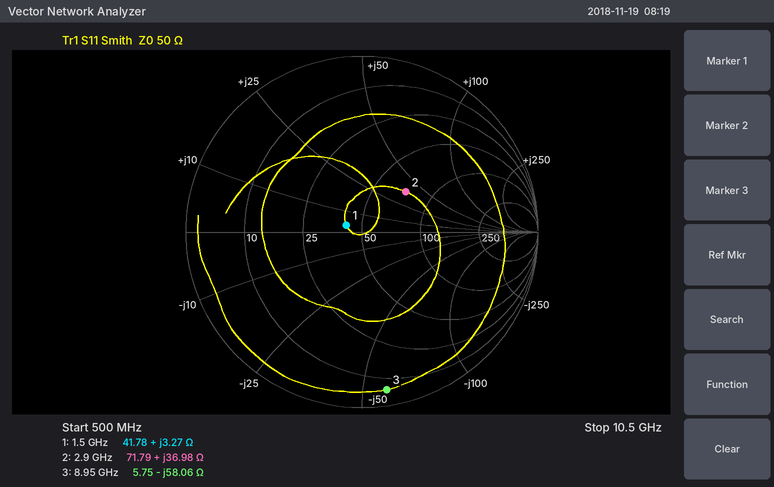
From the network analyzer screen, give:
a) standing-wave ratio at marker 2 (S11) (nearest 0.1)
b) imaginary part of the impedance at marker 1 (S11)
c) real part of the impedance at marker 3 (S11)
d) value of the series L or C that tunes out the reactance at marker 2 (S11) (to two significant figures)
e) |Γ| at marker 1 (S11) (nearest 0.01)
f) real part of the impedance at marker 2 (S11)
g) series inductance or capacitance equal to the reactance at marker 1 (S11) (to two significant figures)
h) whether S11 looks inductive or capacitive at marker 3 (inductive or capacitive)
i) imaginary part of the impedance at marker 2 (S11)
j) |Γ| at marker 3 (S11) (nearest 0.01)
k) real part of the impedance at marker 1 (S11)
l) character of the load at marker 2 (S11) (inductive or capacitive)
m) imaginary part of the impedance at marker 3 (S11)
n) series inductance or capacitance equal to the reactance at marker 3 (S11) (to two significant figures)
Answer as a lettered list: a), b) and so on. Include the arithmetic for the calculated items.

a) 2.0
b) +3.27 Ω
c) 5.75 Ω
d) C = 1/(2π × 2.9 GHz × 36.98 Ω) ≈ 1.5 pF
e) 0.10
f) 71.79 Ω
g) L = 3.27 Ω/(2π × 1.5 GHz) ≈ 347 pH, so 350 pH to two significant figures
h) capacitive
i) +36.98 Ω
j) 0.91
k) 41.78 Ω
l) inductive
m) -58.06 Ω
n) C = 1/(2π × 8.95 GHz × 58.06 Ω) ≈ 306 fF, so 310 fF to two significant figures
